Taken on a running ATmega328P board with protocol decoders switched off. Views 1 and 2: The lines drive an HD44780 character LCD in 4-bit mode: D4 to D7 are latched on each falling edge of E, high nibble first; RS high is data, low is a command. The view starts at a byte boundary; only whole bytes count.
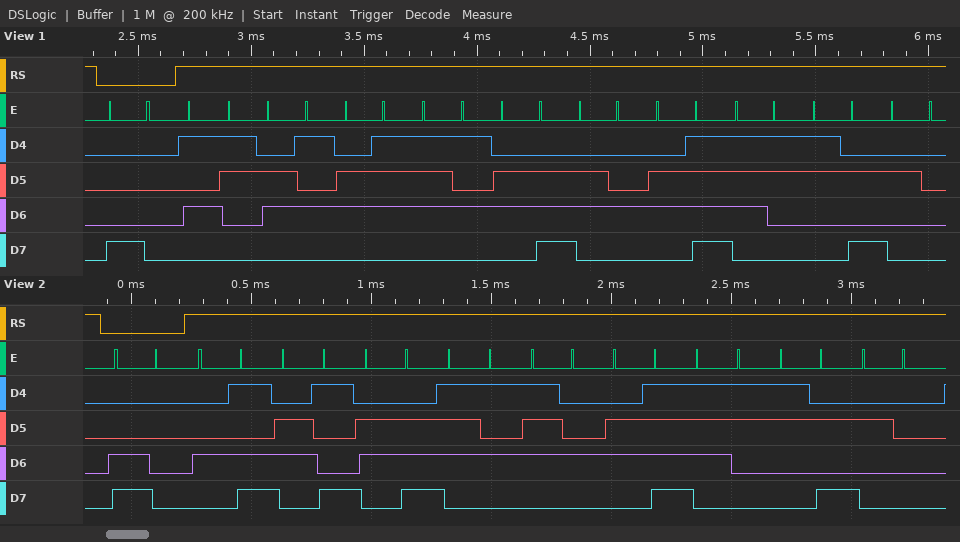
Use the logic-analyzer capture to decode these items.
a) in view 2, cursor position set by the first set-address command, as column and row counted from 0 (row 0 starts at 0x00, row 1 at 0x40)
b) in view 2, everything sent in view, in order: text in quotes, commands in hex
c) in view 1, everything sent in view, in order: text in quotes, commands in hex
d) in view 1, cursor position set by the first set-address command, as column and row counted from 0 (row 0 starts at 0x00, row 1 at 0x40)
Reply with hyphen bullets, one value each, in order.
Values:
- column 0, row 1
- 0xC0 "Minutos: "
- 0x80 "Segundos: "
- column 0, row 0
